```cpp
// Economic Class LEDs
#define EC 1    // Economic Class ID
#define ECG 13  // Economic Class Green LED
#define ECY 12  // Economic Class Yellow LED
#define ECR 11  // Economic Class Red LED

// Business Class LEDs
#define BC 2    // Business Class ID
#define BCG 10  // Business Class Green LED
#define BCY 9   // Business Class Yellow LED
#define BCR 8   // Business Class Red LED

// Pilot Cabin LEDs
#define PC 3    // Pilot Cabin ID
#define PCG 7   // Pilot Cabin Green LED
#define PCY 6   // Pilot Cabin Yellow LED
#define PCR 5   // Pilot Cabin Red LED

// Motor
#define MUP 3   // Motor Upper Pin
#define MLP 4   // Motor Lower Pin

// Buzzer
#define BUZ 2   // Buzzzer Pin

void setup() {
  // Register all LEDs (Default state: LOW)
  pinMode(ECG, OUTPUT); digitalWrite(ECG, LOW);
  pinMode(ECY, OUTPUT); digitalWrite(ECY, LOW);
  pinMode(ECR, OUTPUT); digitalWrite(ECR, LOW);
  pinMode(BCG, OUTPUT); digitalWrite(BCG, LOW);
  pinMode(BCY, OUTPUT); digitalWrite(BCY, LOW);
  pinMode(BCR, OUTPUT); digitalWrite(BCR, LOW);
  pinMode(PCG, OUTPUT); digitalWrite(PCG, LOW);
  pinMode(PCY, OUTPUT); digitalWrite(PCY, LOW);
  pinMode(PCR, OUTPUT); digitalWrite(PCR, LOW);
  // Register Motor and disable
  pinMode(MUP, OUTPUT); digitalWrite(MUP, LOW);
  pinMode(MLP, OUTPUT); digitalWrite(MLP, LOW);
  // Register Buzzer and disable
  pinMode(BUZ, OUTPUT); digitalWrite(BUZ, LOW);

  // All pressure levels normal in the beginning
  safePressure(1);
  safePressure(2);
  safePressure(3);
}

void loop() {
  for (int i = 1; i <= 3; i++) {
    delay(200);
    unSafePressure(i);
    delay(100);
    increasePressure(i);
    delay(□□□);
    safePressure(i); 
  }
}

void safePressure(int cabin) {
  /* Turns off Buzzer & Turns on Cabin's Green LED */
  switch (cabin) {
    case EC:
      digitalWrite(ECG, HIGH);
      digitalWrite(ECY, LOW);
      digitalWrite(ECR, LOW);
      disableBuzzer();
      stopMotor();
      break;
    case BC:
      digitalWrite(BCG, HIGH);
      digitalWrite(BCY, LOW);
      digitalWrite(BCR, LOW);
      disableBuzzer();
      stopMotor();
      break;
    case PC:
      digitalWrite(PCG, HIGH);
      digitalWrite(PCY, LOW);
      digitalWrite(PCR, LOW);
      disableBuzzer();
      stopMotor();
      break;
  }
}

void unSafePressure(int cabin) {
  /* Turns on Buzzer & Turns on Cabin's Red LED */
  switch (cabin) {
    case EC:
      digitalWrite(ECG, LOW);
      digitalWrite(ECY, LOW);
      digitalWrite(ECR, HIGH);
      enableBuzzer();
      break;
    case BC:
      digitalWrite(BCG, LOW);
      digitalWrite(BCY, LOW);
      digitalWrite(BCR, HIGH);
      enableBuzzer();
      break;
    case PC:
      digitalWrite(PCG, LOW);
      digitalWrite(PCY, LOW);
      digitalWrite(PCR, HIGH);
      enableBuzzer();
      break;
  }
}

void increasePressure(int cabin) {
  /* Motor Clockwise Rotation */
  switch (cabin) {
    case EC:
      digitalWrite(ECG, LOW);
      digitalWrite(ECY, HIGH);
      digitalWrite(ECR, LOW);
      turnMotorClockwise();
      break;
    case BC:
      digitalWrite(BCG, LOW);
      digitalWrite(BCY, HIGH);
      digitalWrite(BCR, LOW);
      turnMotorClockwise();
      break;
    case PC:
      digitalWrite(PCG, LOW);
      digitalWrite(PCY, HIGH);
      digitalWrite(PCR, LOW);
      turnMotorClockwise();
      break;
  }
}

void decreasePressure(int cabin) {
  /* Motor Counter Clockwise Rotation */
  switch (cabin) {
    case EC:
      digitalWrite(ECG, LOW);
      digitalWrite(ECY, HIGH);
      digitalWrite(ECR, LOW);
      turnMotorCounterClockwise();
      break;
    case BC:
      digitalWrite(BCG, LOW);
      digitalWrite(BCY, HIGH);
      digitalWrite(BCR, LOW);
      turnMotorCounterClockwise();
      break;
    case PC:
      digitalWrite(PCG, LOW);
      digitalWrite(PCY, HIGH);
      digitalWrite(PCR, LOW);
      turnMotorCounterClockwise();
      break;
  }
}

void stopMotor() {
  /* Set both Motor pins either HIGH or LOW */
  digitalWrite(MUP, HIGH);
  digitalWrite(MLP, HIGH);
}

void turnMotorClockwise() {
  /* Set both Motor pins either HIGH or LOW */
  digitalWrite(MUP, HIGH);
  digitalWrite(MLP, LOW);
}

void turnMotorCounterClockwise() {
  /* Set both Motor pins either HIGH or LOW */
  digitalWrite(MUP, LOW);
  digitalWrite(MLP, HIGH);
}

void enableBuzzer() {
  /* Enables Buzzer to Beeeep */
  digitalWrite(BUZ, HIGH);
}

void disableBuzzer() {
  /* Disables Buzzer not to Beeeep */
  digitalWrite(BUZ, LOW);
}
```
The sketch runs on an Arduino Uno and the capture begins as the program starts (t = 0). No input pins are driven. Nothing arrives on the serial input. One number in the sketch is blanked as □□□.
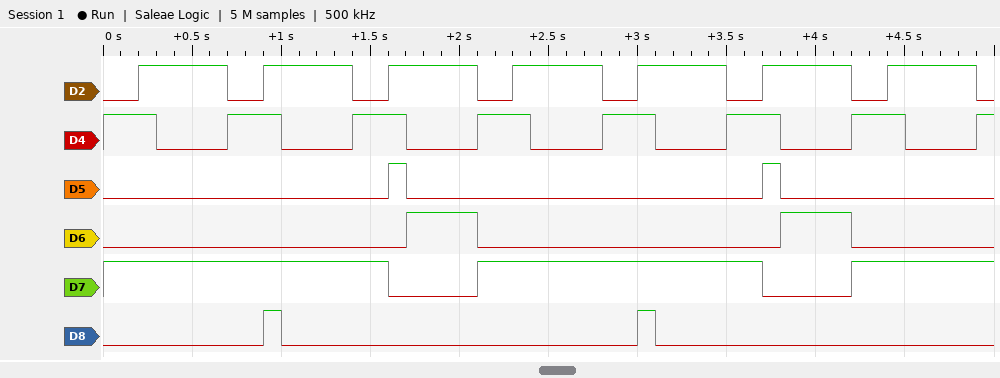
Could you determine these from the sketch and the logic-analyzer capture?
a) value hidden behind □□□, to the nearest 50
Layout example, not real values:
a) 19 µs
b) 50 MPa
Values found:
a) 400
